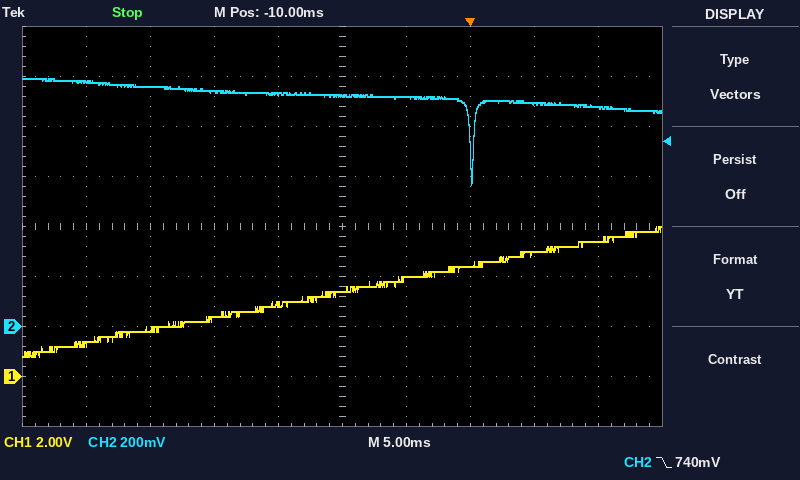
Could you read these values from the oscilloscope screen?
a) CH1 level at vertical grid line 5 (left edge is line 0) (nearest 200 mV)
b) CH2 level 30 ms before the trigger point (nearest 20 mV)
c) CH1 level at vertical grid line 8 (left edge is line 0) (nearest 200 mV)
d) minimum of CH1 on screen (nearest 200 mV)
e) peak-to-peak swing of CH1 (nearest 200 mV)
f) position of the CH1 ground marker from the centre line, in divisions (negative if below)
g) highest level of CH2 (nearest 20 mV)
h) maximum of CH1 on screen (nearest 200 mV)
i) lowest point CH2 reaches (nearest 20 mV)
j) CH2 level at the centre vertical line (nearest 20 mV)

3.4 V
980 mV
5.0 V
800 mV
5.2 V
-3.0 div
1.00 V
6.0 V
560 mV
920 mV
